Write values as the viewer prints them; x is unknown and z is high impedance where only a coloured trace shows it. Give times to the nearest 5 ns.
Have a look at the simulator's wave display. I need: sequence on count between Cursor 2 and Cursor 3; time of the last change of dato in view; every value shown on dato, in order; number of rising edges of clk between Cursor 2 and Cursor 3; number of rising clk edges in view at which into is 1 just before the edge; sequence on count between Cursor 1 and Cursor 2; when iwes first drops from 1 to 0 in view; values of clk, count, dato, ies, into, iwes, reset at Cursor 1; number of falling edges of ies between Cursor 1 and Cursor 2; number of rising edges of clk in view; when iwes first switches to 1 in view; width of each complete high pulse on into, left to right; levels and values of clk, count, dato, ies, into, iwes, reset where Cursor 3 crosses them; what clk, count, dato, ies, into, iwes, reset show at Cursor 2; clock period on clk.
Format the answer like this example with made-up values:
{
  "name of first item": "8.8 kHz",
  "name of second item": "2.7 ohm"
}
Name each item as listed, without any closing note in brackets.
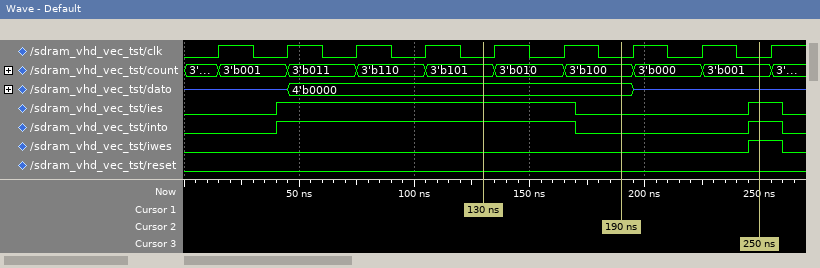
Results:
{
  "sequence on count between Cursor 2 and Cursor 3": "3'b100, 3'b000, 3'b001",
  "time of the last change of dato in view": "195 ns",
  "every value shown on dato, in order": "z, 4'b0000, z",
  "number of rising edges of clk between Cursor 2 and Cursor 3": "2",
  "number of rising clk edges in view at which into is 1 just before the edge": "6",
  "sequence on count between Cursor 1 and Cursor 2": "3'b101, 3'b010, 3'b100",
  "when iwes first drops from 1 to 0 in view": "260 ns",
  "values of clk, count, dato, ies, into, iwes, reset at Cursor 1": "clk=0, count=3'b101, dato=4'b0000, ies=1, into=1, iwes=0, reset=0",
  "number of falling edges of ies between Cursor 1 and Cursor 2": "1",
  "number of rising edges of clk in view": "9",
  "when iwes first switches to 1 in view": "245 ns",
  "width of each complete high pulse on into, left to right": "130 ns, 15 ns",
  "levels and values of clk, count, dato, ies, into, iwes, reset where Cursor 3 crosses them": "clk=0, count=3'b001, dato=z, ies=1, into=1, iwes=1, reset=0",
  "what clk, count, dato, ies, into, iwes, reset show at Cursor 2": "clk=0, count=3'b100, dato=4'b0000, ies=0, into=0, iwes=0, reset=0",
  "clock period on clk": "30 ns"
}
